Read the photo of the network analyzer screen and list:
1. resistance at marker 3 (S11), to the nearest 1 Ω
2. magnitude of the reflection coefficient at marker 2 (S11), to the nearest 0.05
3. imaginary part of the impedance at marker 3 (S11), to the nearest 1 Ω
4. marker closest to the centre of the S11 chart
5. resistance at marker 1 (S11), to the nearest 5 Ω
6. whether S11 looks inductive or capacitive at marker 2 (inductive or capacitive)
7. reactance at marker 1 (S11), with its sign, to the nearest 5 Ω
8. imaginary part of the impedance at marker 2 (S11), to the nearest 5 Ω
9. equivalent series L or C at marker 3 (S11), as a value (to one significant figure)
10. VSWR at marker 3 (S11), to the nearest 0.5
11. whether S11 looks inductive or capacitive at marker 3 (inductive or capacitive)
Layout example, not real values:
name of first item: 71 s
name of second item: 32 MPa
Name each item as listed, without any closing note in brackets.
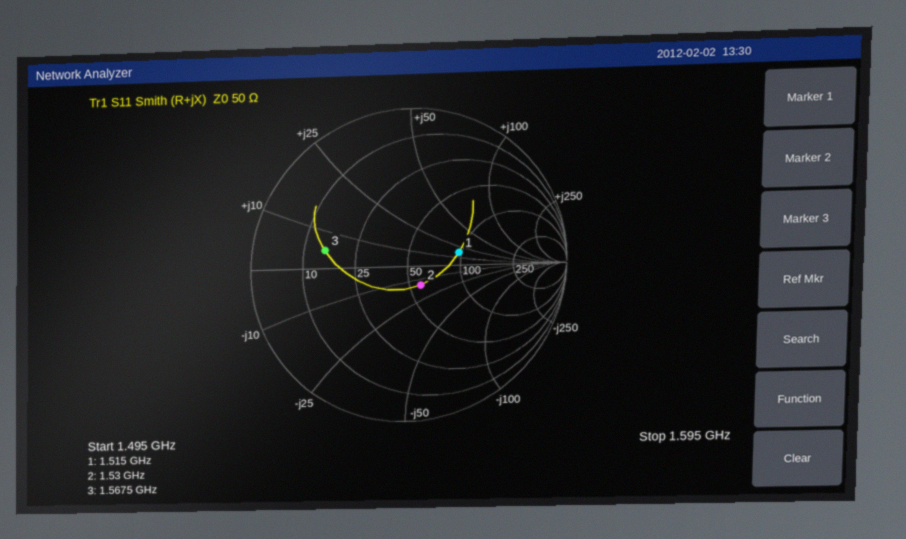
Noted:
resistance at marker 3 (S11), to the nearest 1 Ω: 15 Ω
magnitude of the reflection coefficient at marker 2 (S11), to the nearest 0.05: 0.15
imaginary part of the impedance at marker 3 (S11), to the nearest 1 Ω: +5 Ω
marker closest to the centre of the S11 chart: marker 2
resistance at marker 1 (S11), to the nearest 5 Ω: 95 Ω
whether S11 looks inductive or capacitive at marker 2: capacitive
reactance at marker 1 (S11), with its sign, to the nearest 5 Ω: +15 Ω
imaginary part of the impedance at marker 2 (S11), to the nearest 5 Ω: -15 Ω
equivalent series L or C at marker 3 (S11), as a value: 500 pH
VSWR at marker 3 (S11), to the nearest 0.5: 3.5
whether S11 looks inductive or capacitive at marker 3: inductive
